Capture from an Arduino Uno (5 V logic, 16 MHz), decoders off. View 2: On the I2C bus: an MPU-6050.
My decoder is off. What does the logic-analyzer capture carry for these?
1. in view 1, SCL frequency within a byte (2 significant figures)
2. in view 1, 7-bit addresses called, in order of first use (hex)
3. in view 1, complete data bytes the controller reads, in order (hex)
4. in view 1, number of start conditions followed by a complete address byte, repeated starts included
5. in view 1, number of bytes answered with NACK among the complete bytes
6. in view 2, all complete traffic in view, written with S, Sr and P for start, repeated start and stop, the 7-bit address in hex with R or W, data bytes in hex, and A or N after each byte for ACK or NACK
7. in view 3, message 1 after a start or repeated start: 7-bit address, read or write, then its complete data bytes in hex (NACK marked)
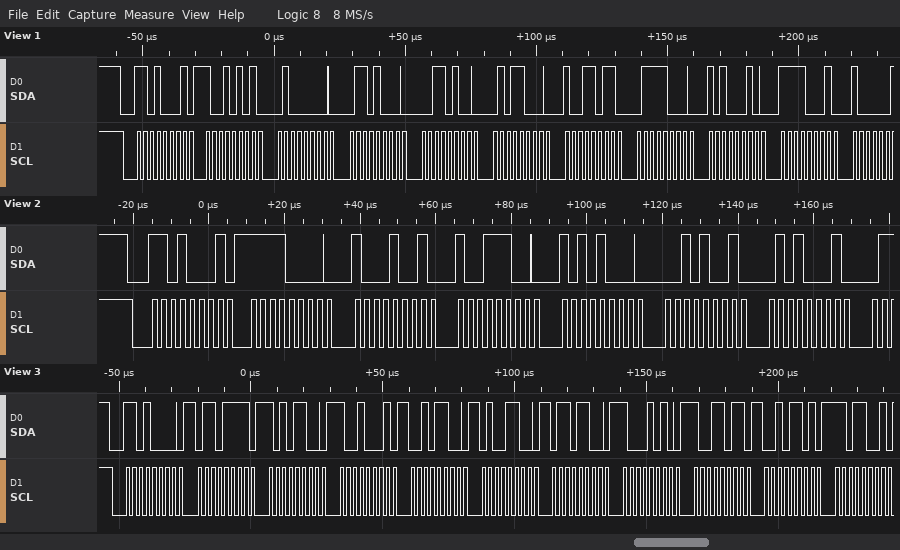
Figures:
400 kHz
0x68
95 40 68 34 58 9B 78 A2 F1
1
0
S 68R A F0 A 89 A 9C A A8 A 29 A 51 A
0x68 write: 6F AC 91 2C 4C 6C 8A 9B 2D D9
